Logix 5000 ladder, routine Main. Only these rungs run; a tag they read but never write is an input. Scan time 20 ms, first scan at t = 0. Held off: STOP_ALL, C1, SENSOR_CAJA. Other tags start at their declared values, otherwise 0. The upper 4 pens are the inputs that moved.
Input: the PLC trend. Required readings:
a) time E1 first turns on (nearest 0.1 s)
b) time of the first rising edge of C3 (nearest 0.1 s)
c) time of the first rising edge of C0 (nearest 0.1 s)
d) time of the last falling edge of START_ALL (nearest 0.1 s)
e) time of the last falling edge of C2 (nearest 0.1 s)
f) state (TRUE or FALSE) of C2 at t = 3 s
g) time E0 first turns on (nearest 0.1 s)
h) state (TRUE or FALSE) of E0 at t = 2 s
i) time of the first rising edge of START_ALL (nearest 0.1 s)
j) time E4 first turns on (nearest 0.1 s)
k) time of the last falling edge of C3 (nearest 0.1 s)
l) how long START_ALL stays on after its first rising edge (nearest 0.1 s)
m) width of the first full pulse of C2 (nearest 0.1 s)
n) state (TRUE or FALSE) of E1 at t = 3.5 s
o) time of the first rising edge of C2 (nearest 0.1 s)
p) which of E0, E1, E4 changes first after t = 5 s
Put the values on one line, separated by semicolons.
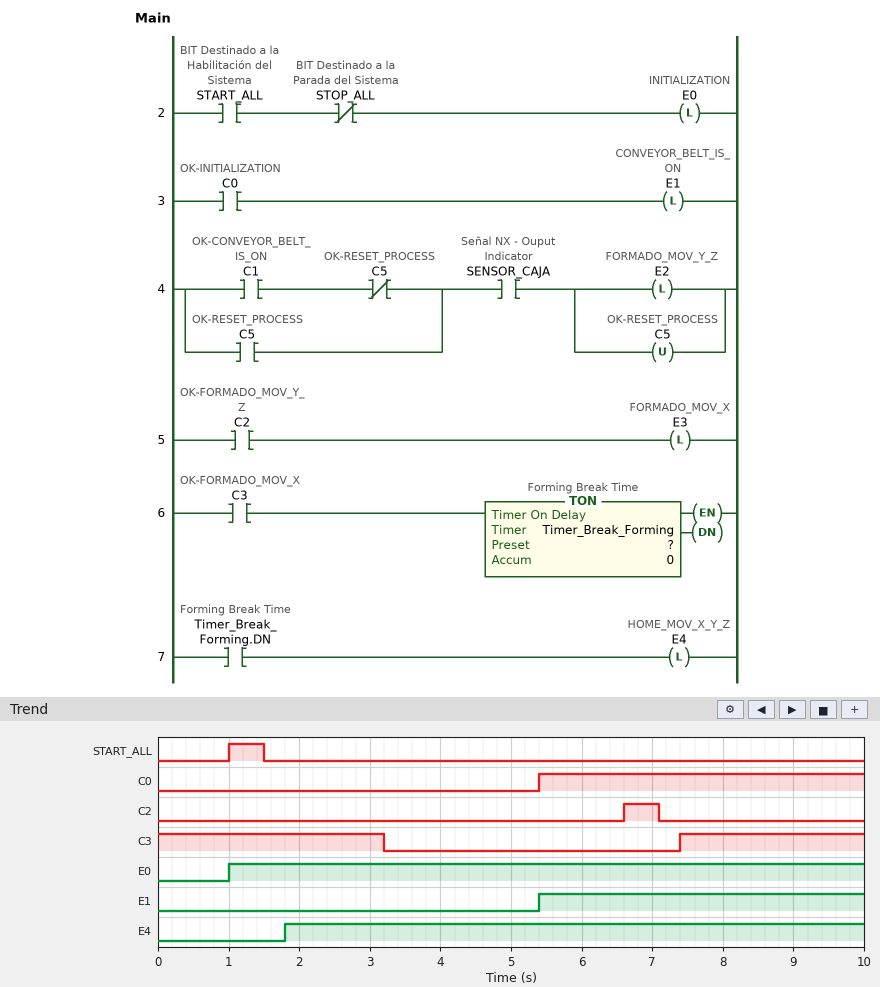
5.4 s; 7.4 s; 5.4 s; 1.5 s; 7.1 s; FALSE; 1.0 s; TRUE; 1.0 s; 1.8 s; 3.2 s; 0.5 s; 0.5 s; FALSE; 6.6 s; E1
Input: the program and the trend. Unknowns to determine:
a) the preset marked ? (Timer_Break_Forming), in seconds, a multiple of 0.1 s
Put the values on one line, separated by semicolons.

1.8 s
